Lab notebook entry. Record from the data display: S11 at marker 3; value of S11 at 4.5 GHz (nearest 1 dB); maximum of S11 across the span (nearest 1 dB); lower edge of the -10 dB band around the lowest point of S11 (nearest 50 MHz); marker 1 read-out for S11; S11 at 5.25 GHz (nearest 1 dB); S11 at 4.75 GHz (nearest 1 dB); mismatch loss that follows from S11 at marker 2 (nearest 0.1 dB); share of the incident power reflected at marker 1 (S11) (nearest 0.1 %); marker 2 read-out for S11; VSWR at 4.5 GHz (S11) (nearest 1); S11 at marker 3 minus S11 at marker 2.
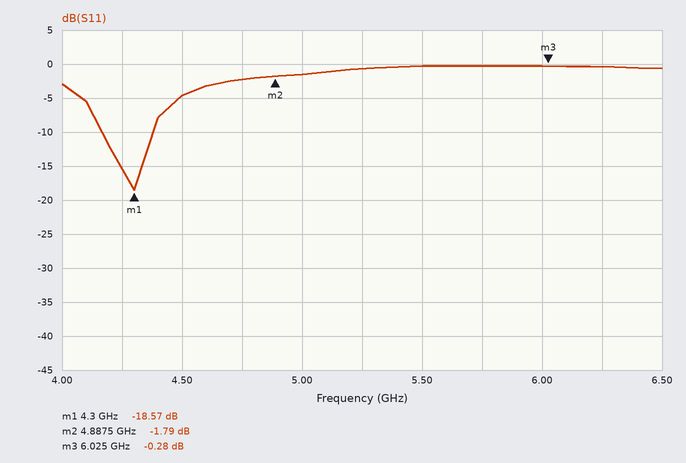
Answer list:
-0.28 dB
-5 dB
0 dB
4.15 GHz
-18.57 dB
-1 dB
-2 dB
4.7 dB
1.4 %
-1.79 dB
4
1.51 dB
